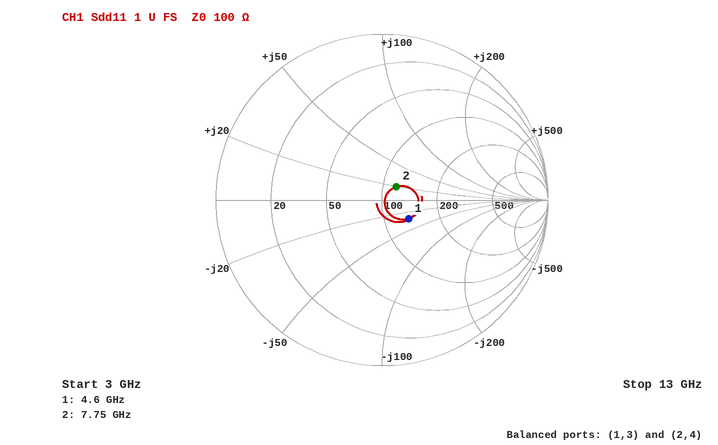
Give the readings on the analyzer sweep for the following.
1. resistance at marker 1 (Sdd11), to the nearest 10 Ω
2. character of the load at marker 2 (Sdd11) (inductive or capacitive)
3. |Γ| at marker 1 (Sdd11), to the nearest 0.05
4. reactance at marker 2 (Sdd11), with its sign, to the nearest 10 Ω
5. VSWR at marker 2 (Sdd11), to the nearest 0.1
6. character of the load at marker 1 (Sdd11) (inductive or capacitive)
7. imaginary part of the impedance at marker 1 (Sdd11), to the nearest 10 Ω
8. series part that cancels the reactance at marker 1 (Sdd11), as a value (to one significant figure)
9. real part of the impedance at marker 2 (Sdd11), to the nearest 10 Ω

130 Ω
inductive
0.20
+20 Ω
1.3
capacitive
-30 Ω
1 nH
120 Ω
